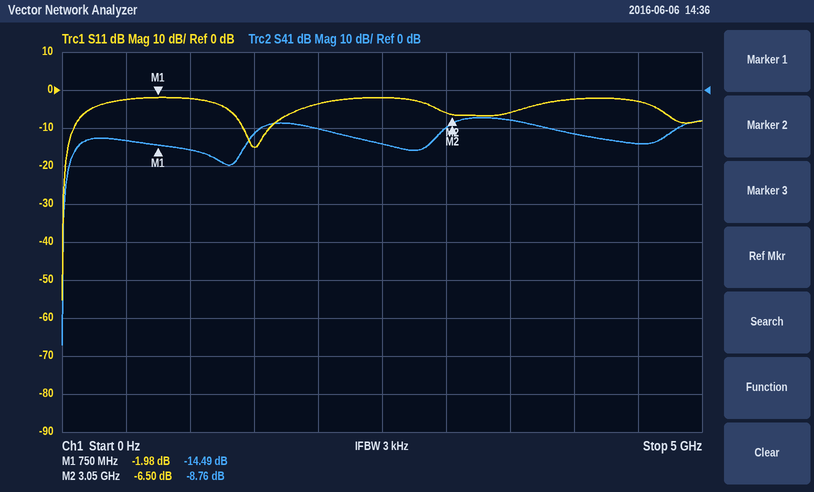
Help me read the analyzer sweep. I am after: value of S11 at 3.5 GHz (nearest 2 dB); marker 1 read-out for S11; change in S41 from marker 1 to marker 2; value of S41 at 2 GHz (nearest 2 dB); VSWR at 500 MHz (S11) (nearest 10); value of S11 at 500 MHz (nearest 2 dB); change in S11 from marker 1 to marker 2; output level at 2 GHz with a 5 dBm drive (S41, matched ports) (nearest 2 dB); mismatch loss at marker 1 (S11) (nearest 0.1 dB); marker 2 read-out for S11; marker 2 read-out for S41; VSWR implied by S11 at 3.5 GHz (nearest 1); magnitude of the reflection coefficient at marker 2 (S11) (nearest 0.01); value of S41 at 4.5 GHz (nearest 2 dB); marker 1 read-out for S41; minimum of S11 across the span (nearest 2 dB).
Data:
-6 dB
-1.98 dB
5.73 dB
-10 dB
10
-2 dB
-4.52 dB
-6 dBm
4.4 dB
-6.50 dB
-8.76 dB
3
0.47
-14 dB
-14.49 dB
-56 dB
